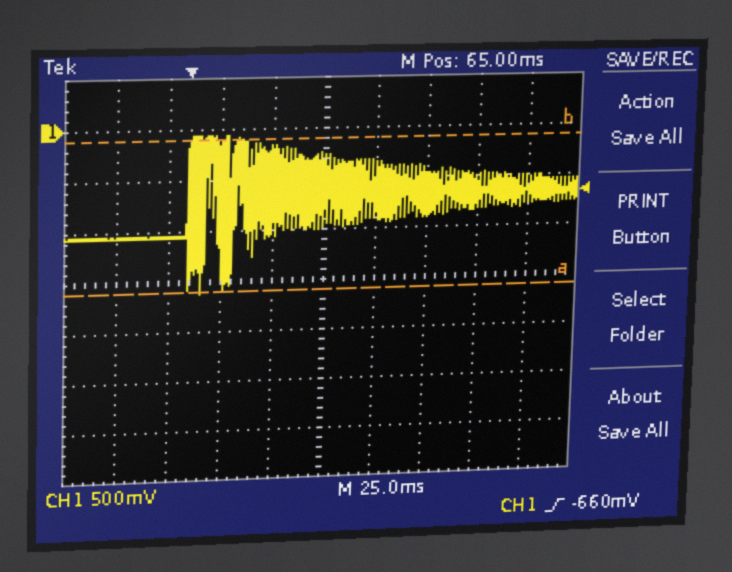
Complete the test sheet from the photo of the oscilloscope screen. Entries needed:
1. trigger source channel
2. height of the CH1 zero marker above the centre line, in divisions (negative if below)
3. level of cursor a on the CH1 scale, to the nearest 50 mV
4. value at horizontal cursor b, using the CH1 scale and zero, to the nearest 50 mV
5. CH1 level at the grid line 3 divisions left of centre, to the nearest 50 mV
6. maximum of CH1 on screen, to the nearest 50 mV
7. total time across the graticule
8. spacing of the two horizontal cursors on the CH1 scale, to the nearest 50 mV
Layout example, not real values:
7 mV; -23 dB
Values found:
CH1; +3.0 div; -1.60 V; -100 mV; -1.05 V; -50 mV; 250 ms; 1.50 V
